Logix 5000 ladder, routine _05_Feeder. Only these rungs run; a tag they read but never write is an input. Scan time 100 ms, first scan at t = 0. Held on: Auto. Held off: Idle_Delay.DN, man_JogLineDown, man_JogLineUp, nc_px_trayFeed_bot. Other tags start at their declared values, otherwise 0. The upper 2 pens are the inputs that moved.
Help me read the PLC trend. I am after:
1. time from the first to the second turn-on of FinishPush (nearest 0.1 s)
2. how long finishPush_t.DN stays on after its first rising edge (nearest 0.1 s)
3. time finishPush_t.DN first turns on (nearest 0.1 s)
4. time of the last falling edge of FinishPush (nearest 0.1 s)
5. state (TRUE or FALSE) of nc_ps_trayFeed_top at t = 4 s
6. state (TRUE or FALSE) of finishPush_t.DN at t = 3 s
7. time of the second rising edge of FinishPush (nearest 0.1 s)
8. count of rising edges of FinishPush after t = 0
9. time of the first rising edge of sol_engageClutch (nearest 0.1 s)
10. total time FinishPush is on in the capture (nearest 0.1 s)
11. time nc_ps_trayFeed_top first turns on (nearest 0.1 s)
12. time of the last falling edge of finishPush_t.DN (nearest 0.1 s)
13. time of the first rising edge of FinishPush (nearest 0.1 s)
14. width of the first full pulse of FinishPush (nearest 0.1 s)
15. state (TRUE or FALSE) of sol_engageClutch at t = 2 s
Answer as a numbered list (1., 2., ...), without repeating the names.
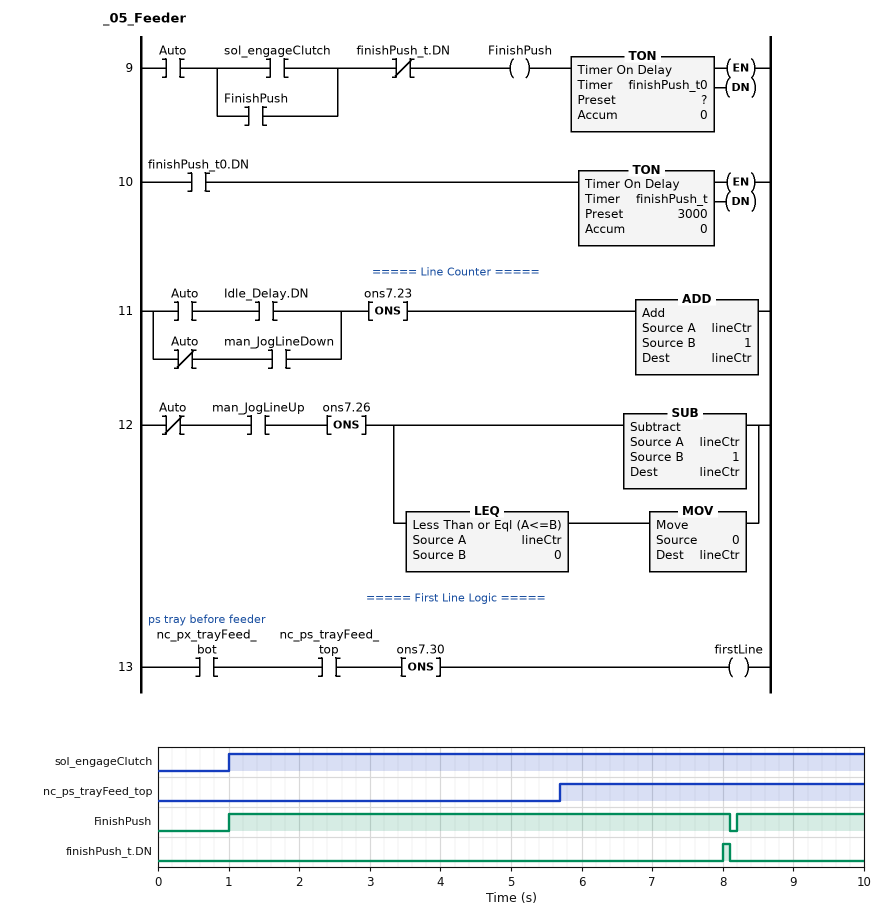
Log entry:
1. 7.2 s
2. 0.1 s
3. 8.0 s
4. 8.1 s
5. FALSE
6. FALSE
7. 8.2 s
8. 2
9. 1.0 s
10. 8.9 s
11. 5.7 s
12. 8.1 s
13. 1.0 s
14. 7.1 s
15. TRUE
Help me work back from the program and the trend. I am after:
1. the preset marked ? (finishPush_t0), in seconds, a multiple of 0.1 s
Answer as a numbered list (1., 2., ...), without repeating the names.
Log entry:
1. 4.0 s
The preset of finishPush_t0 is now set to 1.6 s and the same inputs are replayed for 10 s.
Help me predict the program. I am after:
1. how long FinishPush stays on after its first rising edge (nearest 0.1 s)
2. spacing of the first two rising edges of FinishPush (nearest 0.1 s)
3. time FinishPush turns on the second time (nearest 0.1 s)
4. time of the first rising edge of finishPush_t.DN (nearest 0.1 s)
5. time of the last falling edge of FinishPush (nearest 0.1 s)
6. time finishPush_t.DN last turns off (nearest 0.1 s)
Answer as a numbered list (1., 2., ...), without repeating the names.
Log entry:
1. 4.7 s
2. 4.8 s
3. 5.8 s
4. 5.6 s
5. 5.7 s
6. 5.7 s
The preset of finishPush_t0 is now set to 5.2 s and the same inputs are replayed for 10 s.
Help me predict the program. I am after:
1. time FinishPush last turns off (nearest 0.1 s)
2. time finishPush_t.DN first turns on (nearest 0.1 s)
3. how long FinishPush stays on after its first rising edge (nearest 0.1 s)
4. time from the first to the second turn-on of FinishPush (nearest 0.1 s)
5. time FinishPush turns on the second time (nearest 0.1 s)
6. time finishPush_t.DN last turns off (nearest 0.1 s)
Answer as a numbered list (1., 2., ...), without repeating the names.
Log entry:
1. 9.3 s
2. 9.2 s
3. 8.3 s
4. 8.4 s
5. 9.4 s
6. 9.3 s
